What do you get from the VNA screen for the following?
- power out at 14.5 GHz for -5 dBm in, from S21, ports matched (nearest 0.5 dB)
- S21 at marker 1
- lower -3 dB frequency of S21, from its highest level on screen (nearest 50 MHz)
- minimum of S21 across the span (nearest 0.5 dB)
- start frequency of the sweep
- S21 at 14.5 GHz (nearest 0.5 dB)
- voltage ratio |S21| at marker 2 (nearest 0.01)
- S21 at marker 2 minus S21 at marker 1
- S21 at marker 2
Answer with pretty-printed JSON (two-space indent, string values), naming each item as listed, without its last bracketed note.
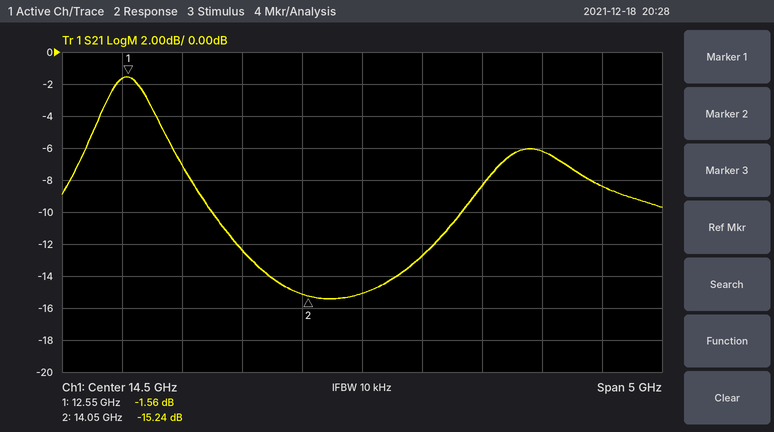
{
  "power out at 14.5 GHz for -5 dBm in, from S21, ports matched": "-20.0 dBm",
  "S21 at marker 1": "-1.56 dB",
  "lower -3 dB frequency of S21, from its highest level on screen": "12.30 GHz",
  "minimum of S21 across the span": "-15.5 dB",
  "start frequency of the sweep": "12 GHz",
  "S21 at 14.5 GHz": "-15.0 dB",
  "voltage ratio |S21| at marker 2": "0.17",
  "S21 at marker 2 minus S21 at marker 1": "-13.68 dB",
  "S21 at marker 2": "-15.24 dB"
}
